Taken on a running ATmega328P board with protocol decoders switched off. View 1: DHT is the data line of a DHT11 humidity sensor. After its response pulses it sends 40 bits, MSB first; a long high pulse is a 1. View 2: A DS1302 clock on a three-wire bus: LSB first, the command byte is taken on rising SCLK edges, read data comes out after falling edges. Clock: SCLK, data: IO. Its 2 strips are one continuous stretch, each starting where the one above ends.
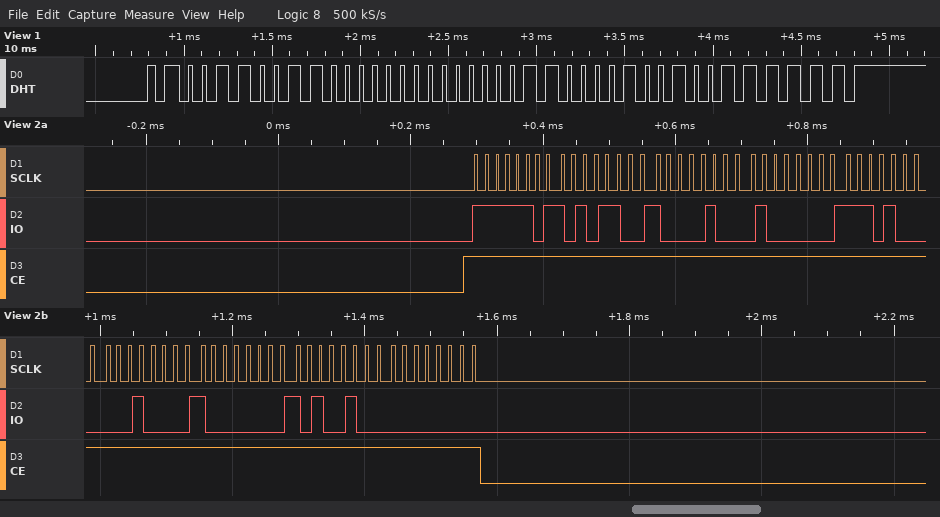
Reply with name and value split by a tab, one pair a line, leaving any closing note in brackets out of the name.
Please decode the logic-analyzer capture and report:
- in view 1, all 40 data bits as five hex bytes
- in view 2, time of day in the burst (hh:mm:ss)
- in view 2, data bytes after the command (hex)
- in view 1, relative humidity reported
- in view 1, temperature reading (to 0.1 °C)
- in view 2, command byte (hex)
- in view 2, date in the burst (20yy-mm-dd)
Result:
in view 1, all 40 data bits as five hex bytes	33 00 03 09 3F
in view 2, time of day in the burst	02:21:35
in view 2, data bytes after the command	35 21 02 17 08 01 25 00
in view 1, relative humidity reported	51 %
in view 1, temperature reading	3.9 °C
in view 2, command byte	0xBF
in view 2, date in the burst	2025-08-17
